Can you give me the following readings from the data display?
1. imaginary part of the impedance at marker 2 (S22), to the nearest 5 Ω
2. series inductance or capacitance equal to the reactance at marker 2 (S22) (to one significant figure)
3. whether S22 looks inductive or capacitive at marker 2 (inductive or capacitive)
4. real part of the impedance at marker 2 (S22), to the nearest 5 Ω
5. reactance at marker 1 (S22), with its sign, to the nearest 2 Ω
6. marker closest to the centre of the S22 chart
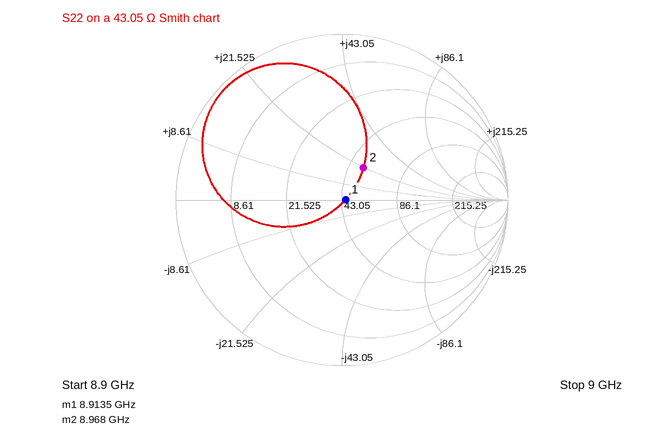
+20 Ω
400 pH
inductive
50 Ω
0 Ω
marker 1
